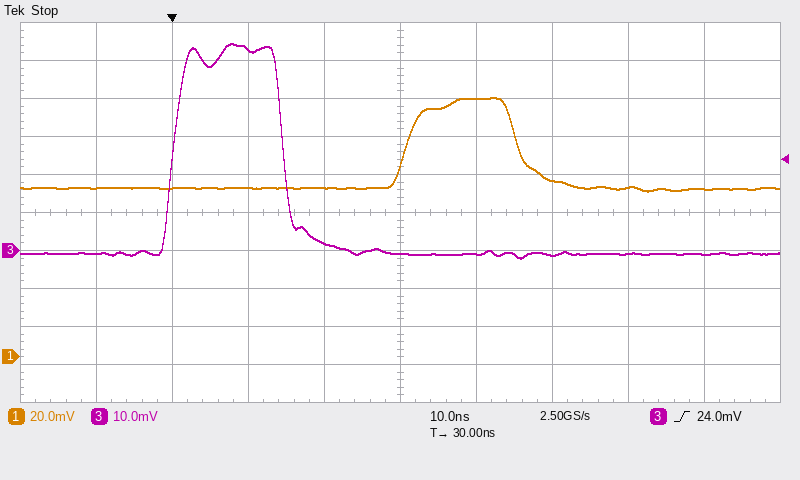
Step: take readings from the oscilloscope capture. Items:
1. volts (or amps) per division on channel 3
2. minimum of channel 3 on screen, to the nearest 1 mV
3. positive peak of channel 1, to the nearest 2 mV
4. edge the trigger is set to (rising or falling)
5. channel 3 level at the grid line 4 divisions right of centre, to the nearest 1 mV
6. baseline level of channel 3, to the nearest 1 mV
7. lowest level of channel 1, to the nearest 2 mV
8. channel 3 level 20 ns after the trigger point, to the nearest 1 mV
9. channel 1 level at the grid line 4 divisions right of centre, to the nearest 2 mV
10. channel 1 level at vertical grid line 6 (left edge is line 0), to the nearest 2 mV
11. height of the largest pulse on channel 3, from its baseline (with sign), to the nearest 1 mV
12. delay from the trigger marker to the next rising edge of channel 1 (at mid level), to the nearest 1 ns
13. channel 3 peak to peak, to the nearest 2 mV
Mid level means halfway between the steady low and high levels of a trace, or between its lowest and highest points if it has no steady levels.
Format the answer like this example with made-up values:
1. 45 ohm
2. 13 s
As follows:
1. 10 mV
2. -2 mV
3. 136 mV
4. rising
5. -1 mV
6. -1 mV
7. 88 mV
8. 2 mV
9. 88 mV
10. 136 mV
11. +55 mV
12. 31 ns
13. 56 mV
